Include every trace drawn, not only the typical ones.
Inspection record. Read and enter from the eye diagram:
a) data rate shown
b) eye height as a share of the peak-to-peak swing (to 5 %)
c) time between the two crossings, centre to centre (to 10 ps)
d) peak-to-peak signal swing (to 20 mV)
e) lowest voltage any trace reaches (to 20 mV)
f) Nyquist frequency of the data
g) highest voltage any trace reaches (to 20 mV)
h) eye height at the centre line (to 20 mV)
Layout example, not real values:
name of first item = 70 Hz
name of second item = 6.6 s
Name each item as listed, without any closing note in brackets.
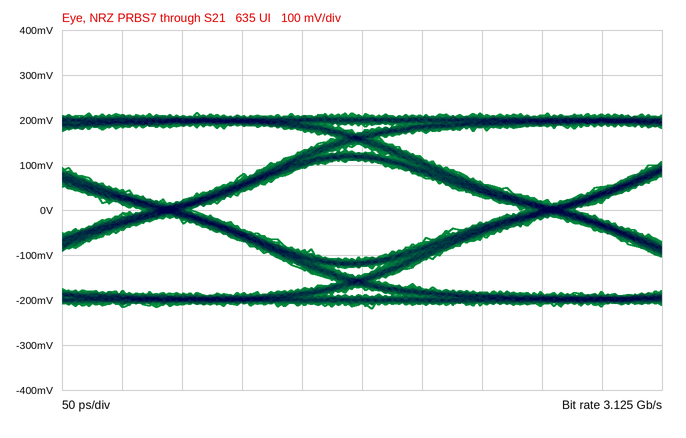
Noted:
data rate shown = 3.125 Gb/s
eye height as a share of the peak-to-peak swing = 50 %
time between the two crossings, centre to centre = 320 ps
peak-to-peak signal swing = 440 mV
lowest voltage any trace reaches = -220 mV
Nyquist frequency of the data = 1.5625 GHz
highest voltage any trace reaches = 220 mV
eye height at the centre line = 220 mV
